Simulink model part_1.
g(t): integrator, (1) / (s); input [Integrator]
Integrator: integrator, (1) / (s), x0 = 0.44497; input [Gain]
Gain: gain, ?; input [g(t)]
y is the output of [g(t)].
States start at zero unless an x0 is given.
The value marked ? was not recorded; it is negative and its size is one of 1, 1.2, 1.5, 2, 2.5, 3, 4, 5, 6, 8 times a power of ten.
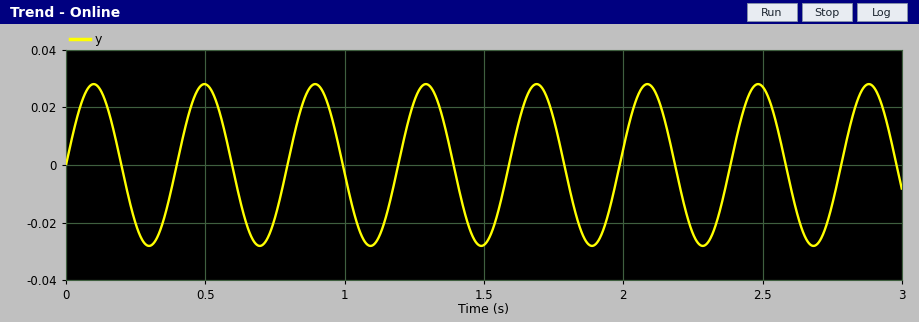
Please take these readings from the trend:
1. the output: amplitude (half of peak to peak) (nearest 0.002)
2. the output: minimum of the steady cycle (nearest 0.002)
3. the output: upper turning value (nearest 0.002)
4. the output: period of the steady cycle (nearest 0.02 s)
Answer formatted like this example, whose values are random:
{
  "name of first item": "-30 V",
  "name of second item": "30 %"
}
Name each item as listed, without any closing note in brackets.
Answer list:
{
  "the output: amplitude (half of peak to peak)": "0.028",
  "the output: minimum of the steady cycle": "-0.028",
  "the output: upper turning value": "0.028",
  "the output: period of the steady cycle": "0.40 s"
}
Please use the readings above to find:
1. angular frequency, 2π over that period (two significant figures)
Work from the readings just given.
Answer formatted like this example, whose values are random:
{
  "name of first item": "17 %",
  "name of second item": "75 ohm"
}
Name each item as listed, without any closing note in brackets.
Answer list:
{
  "angular frequency, 2π over that period": "16 rad/s"
}
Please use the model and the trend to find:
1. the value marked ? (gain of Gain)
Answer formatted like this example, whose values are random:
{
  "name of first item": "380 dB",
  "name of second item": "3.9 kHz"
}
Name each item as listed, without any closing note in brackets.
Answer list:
{
  "the value marked ?": "-250"
}
